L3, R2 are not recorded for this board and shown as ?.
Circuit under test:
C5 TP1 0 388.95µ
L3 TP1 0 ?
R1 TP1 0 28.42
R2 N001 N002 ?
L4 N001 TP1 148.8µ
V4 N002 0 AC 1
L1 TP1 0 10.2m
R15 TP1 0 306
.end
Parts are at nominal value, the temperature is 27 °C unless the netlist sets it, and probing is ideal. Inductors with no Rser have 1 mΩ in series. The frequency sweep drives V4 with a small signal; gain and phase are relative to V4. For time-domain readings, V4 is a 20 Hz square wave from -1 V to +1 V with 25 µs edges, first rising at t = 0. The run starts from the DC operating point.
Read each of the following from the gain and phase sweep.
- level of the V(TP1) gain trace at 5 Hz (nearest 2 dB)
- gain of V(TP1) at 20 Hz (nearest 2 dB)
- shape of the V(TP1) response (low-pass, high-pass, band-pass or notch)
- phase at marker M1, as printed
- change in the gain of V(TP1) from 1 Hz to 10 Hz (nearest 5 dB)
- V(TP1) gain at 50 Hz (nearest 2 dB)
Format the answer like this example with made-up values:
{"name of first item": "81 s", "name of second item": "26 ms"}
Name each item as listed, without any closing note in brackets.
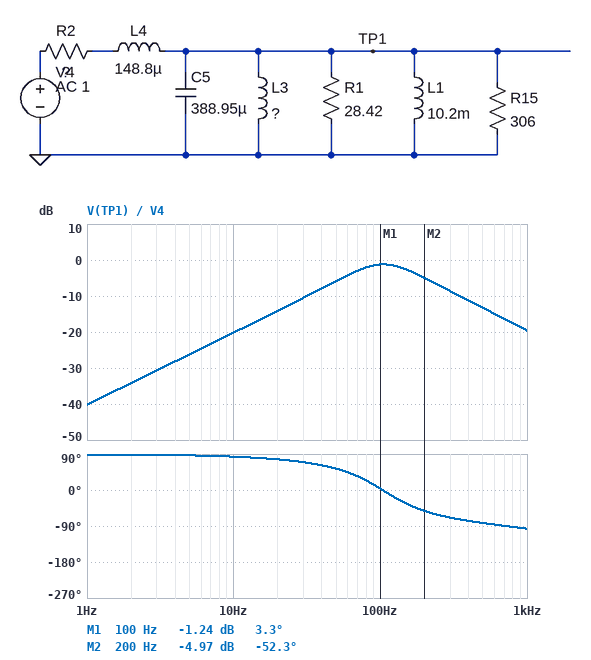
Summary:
{"level of the V(TP1) gain trace at 5 Hz": "-26 dB", "gain of V(TP1) at 20 Hz": "-14 dB", "shape of the V(TP1) response": "band-pass", "phase at marker M1, as printed": "3.3 deg", "change in the gain of V(TP1) from 1 Hz to 10 Hz": "20 dB", "V(TP1) gain at 50 Hz": "-6 dB"}
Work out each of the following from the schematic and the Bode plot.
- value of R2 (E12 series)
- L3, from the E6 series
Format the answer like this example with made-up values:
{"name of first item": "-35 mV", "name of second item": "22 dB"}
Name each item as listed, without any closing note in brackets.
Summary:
{"value of R2": "3.9 Ω", "L3, from the E6 series": "15 mH"}
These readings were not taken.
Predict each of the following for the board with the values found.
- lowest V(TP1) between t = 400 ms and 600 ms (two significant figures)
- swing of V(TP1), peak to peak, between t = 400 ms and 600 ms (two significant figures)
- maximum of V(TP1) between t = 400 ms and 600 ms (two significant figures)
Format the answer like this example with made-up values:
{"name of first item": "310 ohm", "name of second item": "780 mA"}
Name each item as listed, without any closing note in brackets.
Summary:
{"lowest V(TP1) between t = 400 ms and 600 ms": "-1.0 V", "swing of V(TP1), peak to peak, between t = 400 ms and 600 ms": "2.1 V", "maximum of V(TP1) between t = 400 ms and 600 ms": "1.0 V"}
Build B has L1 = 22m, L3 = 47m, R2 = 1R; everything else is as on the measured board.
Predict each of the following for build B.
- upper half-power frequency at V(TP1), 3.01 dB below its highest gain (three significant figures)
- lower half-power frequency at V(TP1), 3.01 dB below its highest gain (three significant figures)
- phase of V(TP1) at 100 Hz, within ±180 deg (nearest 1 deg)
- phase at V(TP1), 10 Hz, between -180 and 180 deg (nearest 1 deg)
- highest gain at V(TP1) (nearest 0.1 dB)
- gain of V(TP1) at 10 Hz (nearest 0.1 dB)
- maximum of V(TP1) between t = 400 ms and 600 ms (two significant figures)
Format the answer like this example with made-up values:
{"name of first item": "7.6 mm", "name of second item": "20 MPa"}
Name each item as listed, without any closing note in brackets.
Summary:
{"upper half-power frequency at V(TP1), 3.01 dB below its highest gain": "588 Hz", "lower half-power frequency at V(TP1), 3.01 dB below its highest gain": "10.2 Hz", "phase of V(TP1) at 100 Hz, within ±180 deg": "-8 deg", "phase at V(TP1), 10 Hz, between -180 and 180 deg": "45 deg", "highest gain at V(TP1)": "-0.3 dB", "gain of V(TP1) at 10 Hz": "-3.4 dB", "maximum of V(TP1) between t = 400 ms and 600 ms": "1.6 V"}
